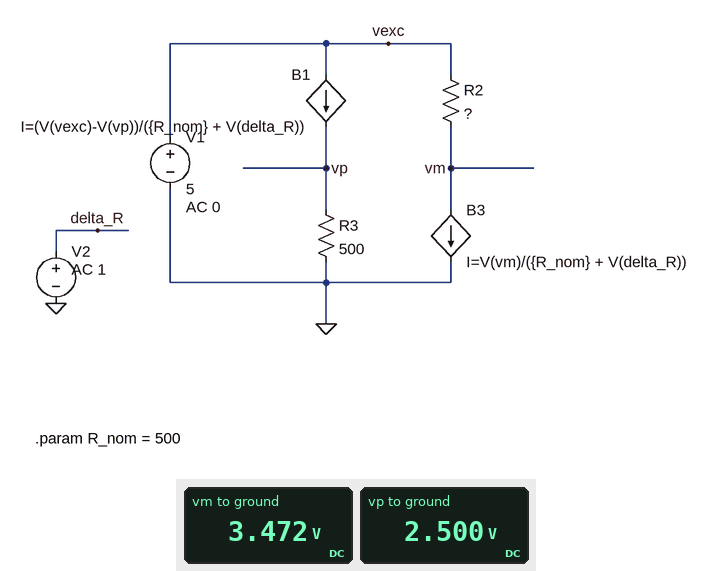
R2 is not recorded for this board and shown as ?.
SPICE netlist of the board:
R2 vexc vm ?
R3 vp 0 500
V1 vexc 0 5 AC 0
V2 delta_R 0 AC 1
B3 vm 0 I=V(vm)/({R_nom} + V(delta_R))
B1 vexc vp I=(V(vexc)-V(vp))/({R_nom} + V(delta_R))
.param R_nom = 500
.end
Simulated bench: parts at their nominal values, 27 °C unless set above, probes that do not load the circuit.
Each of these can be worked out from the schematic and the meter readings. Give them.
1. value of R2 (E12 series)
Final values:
220 Ω
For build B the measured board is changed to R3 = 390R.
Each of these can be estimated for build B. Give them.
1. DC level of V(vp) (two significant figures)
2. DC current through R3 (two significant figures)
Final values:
2.2 V
5.6 mA
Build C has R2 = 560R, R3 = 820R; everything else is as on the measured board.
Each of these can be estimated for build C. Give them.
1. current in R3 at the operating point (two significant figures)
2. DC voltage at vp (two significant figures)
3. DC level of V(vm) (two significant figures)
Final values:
3.8 mA
3.1 V
2.4 V
